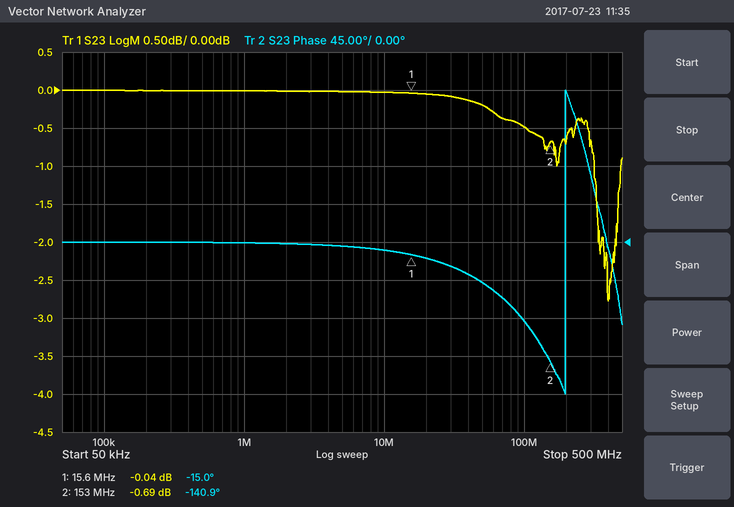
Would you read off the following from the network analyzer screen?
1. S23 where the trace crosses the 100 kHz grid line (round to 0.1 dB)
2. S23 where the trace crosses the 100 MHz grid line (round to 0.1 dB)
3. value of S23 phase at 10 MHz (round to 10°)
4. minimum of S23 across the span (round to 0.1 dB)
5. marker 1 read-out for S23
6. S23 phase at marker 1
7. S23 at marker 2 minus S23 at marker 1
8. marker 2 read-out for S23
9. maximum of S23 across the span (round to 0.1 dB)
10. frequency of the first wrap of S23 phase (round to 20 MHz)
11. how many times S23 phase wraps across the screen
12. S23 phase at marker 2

0.0 dB
-0.5 dB
-10°
-2.8 dB
-0.04 dB
-15.0°
-0.65 dB
-0.69 dB
0.0 dB
200 MHz
1
-140.9°
